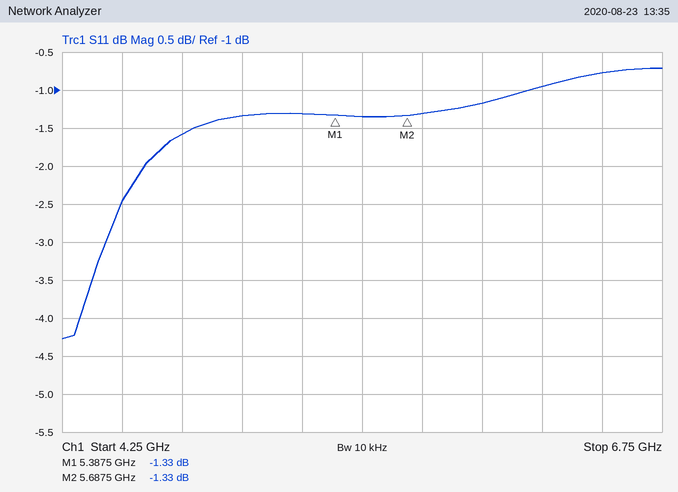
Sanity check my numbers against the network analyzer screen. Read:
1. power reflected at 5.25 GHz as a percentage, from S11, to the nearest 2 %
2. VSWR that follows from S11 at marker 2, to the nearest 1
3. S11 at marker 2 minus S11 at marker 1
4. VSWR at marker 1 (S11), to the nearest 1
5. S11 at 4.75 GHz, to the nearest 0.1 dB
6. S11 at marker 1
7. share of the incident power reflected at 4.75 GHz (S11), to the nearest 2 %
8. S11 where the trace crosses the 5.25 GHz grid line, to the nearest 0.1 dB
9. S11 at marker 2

74 %
13
0.00 dB
13
-1.6 dB
-1.33 dB
70 %
-1.3 dB
-1.33 dB
